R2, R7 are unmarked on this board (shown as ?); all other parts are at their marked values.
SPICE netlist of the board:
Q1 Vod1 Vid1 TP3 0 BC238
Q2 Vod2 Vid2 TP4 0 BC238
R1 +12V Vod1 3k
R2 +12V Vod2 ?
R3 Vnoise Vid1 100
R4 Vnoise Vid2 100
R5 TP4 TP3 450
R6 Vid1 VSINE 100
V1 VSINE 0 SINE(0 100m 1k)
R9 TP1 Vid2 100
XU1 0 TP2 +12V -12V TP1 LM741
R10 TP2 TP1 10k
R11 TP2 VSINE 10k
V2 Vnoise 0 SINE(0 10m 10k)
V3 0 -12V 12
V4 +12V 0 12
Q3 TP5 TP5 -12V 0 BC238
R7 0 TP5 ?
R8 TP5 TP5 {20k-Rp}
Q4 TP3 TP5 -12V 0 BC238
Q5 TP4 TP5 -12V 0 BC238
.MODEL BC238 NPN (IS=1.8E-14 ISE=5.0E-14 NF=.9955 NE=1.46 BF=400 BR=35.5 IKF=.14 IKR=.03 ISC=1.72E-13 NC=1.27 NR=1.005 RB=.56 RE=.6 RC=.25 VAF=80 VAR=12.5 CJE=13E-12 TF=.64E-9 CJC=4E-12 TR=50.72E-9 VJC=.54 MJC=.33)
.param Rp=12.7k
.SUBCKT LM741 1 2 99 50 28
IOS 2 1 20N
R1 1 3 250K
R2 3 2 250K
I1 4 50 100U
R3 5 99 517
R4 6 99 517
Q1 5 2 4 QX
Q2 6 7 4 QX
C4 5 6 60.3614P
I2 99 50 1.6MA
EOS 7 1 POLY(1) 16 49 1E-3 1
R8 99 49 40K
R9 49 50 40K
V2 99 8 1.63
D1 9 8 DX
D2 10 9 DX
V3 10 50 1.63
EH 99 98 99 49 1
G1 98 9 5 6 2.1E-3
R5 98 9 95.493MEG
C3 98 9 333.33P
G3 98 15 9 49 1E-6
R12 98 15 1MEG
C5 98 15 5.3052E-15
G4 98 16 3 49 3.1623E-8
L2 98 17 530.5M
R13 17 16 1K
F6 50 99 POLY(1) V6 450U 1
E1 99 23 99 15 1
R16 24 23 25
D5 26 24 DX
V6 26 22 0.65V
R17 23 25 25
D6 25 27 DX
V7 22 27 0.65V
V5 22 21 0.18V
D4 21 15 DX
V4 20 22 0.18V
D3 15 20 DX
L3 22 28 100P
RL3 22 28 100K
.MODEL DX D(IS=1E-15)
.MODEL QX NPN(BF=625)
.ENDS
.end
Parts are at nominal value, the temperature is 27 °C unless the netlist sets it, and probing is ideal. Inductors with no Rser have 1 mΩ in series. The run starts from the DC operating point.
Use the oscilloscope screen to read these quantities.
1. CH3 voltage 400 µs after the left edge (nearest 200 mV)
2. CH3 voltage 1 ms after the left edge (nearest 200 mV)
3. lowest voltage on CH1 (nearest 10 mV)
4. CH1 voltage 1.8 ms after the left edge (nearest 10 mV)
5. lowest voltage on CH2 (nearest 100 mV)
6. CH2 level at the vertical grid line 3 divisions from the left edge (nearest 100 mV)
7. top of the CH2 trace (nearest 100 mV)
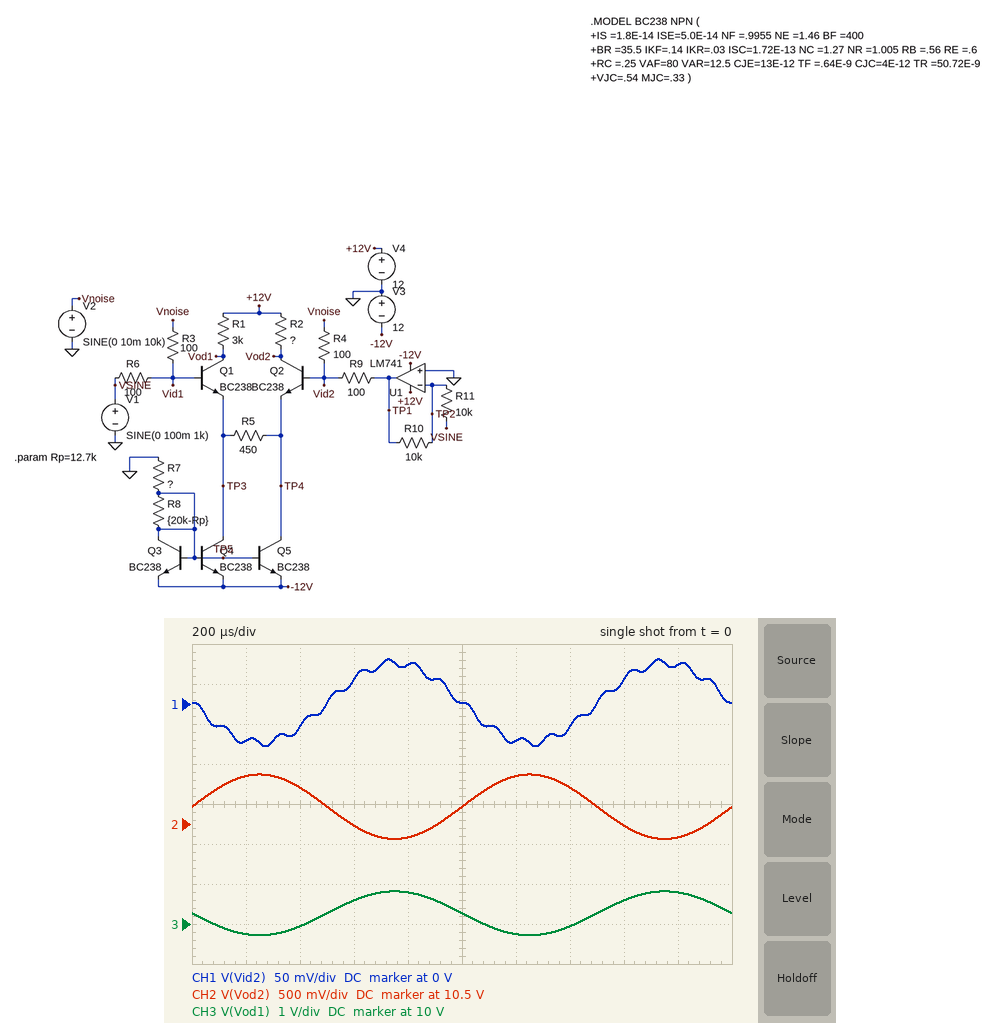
10.0 V
10.2 V
-50 mV
50 mV
10.3 V
10.5 V
11.1 V
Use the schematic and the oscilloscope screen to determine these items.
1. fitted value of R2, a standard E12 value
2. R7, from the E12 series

2.2 kΩ
22 kΩ
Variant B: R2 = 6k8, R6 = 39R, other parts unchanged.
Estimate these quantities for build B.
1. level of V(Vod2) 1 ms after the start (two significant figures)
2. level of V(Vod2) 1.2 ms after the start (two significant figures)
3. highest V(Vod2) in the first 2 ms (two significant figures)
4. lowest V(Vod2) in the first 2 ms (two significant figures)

8.0 V
9.5 V
9.6 V
6.5 V
